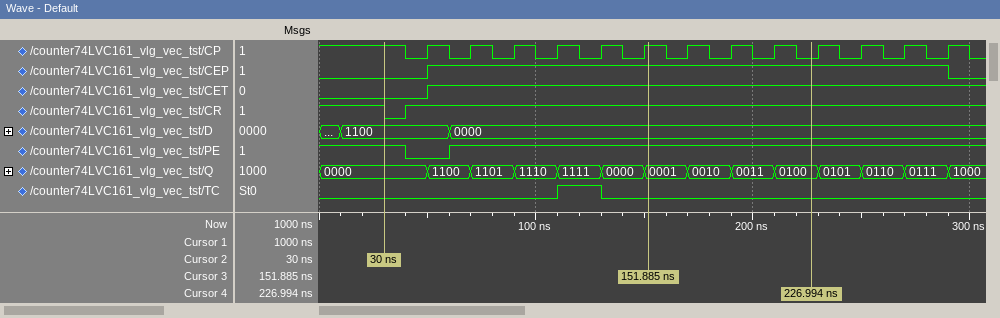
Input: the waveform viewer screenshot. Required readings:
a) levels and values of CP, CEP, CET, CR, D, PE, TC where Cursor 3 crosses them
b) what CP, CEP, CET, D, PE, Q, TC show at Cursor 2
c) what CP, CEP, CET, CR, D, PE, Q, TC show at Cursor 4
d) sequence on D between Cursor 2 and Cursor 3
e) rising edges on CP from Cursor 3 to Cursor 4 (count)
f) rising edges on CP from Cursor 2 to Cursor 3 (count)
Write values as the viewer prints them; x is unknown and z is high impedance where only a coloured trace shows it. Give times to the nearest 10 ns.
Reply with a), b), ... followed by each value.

a) CP=1, CEP=1, CET=1, CR=1, D=0000, PE=1, TC=0
b) CP=1, CEP=0, CET=0, D=1100, PE=1, Q=0000, TC=0
c) CP=0, CEP=1, CET=1, CR=1, D=0000, PE=1, Q=0100, TC=0
d) 1100, 0000
e) 3
f) 6
